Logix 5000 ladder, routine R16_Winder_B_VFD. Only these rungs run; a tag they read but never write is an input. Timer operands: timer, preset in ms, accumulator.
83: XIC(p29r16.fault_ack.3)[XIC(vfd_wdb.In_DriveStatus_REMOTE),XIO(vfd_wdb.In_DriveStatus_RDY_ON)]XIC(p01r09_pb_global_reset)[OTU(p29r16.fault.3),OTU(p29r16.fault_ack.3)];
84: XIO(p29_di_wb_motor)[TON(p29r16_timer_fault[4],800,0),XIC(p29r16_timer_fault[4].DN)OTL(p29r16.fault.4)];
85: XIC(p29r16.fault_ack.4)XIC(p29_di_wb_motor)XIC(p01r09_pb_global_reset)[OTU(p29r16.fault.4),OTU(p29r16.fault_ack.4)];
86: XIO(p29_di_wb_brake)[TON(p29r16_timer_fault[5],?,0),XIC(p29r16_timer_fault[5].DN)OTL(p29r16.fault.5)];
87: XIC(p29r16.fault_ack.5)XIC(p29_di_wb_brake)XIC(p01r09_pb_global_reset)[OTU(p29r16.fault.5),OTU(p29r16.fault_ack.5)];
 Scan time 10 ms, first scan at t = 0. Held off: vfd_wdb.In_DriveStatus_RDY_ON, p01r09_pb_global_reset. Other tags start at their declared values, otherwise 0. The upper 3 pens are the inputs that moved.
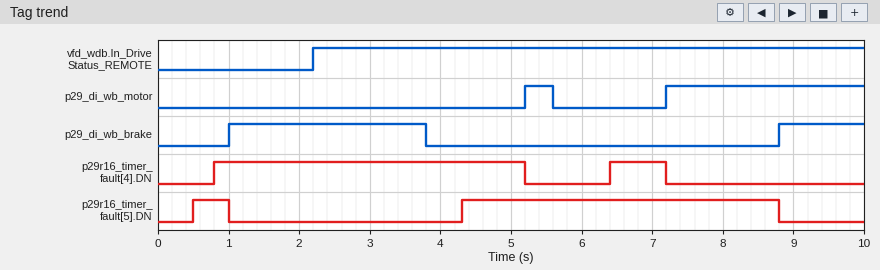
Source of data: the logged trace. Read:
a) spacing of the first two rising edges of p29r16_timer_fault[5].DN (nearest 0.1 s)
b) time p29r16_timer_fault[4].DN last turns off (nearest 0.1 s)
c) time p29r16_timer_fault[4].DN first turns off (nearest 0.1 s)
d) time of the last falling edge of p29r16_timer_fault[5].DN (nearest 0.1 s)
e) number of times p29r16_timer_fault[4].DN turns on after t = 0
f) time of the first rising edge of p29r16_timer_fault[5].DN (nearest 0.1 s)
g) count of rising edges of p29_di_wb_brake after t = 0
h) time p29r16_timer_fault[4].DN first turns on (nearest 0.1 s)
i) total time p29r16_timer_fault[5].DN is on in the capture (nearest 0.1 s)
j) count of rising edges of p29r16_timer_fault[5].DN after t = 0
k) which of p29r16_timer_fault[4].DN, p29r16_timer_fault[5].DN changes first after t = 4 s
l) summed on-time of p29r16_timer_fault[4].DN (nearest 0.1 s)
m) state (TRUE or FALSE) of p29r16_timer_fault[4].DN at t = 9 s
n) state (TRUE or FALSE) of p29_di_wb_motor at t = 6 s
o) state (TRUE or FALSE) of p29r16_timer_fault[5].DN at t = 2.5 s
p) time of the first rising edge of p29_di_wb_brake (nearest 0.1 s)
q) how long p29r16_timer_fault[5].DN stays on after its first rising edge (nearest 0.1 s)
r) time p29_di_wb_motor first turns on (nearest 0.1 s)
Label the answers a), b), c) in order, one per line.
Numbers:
a) 3.8 s
b) 7.2 s
c) 5.2 s
d) 8.8 s
e) 2
f) 0.5 s
g) 2
h) 0.8 s
i) 5.0 s
j) 2
k) p29r16_timer_fault[5].DN
l) 5.2 s
m) FALSE
n) FALSE
o) FALSE
p) 1.0 s
q) 0.5 s
r) 5.2 s
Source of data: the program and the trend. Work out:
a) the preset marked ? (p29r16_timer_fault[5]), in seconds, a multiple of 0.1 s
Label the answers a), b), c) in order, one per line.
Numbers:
a) 0.5 s
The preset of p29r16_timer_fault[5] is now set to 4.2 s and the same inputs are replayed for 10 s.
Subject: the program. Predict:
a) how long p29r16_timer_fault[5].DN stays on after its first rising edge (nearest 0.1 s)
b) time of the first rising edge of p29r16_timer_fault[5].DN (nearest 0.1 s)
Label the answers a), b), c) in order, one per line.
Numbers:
a) 0.8 s
b) 8.0 s
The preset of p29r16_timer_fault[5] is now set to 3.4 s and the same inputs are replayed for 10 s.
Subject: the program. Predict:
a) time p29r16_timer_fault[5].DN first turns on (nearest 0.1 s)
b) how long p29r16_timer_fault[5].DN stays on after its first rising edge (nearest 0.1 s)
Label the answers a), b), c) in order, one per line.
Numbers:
a) 7.2 s
b) 1.6 s
